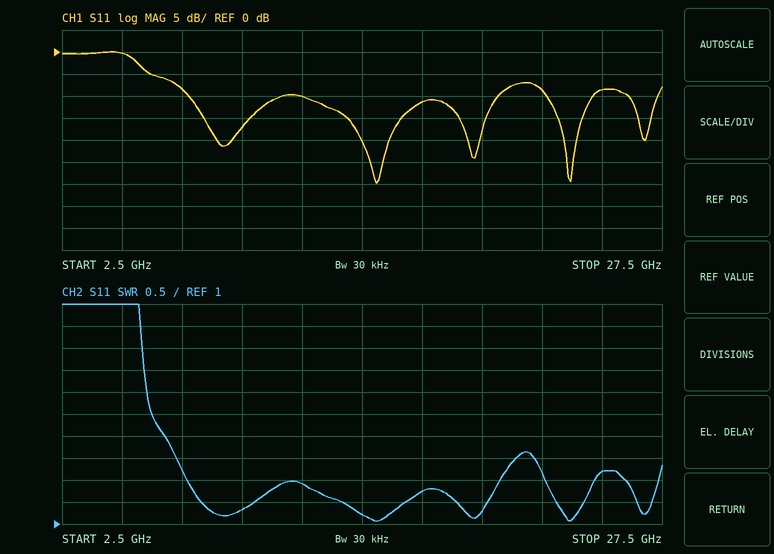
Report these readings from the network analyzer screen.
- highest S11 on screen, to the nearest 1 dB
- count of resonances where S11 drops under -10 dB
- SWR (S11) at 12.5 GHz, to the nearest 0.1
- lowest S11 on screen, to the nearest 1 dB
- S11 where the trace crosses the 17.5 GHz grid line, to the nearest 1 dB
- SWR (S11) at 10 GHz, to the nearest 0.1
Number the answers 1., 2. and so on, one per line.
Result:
1. 0 dB
2. 5
3. 1.9
4. -30 dB
5. -11 dB
6. 1.3
